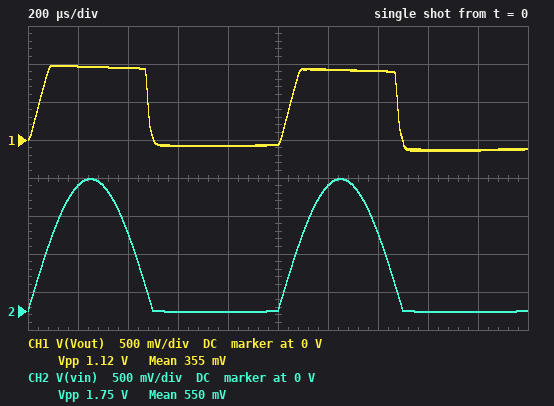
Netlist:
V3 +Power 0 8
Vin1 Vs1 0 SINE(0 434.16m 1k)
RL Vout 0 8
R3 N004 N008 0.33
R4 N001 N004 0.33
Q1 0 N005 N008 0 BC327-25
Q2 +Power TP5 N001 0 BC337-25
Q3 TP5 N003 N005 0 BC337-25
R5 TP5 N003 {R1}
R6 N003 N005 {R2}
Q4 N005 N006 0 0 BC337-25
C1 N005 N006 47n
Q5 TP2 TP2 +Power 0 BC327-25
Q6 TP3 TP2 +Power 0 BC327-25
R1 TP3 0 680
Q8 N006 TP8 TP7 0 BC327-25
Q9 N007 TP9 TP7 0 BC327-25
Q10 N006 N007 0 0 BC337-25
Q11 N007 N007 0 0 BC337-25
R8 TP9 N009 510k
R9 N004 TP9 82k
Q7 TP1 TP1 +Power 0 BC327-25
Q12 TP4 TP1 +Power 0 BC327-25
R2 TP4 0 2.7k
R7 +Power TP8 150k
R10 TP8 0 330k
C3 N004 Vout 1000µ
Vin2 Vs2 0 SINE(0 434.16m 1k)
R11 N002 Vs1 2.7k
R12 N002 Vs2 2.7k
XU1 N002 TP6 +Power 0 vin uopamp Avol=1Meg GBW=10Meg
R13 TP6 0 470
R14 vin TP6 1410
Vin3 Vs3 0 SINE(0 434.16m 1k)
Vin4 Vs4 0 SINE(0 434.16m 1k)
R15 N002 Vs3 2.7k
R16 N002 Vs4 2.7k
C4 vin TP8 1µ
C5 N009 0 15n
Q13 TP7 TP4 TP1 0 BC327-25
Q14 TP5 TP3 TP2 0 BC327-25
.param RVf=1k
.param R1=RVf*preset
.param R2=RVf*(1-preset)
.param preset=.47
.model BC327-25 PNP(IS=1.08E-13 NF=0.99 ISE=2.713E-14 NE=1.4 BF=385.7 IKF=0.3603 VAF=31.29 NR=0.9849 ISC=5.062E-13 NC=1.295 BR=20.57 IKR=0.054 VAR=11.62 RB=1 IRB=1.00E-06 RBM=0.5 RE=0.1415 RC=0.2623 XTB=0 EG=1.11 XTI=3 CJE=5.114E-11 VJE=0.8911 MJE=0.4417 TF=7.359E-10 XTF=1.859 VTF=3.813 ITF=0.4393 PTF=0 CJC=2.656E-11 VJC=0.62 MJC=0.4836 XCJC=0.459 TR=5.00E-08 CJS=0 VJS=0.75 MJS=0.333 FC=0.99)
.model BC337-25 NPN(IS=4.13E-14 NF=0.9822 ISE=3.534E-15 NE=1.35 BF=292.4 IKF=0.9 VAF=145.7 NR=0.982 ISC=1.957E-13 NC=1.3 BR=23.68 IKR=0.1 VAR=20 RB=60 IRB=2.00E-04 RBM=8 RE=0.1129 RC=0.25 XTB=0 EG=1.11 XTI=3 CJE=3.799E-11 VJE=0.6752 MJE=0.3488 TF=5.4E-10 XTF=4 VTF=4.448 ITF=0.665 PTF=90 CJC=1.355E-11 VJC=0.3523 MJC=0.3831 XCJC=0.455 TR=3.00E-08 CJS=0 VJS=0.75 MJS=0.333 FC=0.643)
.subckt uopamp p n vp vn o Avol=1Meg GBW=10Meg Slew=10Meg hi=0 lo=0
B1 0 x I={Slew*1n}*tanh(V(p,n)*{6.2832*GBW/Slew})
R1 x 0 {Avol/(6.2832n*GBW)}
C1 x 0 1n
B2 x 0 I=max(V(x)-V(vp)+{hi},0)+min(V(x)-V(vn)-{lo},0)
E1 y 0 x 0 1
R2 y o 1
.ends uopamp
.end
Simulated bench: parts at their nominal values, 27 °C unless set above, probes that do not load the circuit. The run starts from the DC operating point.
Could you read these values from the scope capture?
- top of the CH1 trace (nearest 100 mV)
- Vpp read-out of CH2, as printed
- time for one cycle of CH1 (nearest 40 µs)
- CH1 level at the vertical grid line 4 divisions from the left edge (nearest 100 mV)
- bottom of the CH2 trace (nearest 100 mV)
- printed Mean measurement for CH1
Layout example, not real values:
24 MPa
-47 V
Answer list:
1.0 V
1.75 V
1.00 ms
-100 mV
0 V
355 mV
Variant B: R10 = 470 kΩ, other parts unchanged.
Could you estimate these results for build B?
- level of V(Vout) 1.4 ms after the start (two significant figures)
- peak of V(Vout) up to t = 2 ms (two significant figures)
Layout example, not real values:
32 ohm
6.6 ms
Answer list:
410 mV
440 mV
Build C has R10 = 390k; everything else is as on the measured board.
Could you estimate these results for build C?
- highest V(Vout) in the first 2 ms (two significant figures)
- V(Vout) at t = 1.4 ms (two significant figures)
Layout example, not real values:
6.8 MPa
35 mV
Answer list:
710 mV
660 mV
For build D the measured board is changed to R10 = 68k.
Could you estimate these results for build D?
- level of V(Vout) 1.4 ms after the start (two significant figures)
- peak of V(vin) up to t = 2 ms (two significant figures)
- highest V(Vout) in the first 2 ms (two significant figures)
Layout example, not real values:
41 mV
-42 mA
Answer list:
1.1 V
1.7 V
2.0 V
